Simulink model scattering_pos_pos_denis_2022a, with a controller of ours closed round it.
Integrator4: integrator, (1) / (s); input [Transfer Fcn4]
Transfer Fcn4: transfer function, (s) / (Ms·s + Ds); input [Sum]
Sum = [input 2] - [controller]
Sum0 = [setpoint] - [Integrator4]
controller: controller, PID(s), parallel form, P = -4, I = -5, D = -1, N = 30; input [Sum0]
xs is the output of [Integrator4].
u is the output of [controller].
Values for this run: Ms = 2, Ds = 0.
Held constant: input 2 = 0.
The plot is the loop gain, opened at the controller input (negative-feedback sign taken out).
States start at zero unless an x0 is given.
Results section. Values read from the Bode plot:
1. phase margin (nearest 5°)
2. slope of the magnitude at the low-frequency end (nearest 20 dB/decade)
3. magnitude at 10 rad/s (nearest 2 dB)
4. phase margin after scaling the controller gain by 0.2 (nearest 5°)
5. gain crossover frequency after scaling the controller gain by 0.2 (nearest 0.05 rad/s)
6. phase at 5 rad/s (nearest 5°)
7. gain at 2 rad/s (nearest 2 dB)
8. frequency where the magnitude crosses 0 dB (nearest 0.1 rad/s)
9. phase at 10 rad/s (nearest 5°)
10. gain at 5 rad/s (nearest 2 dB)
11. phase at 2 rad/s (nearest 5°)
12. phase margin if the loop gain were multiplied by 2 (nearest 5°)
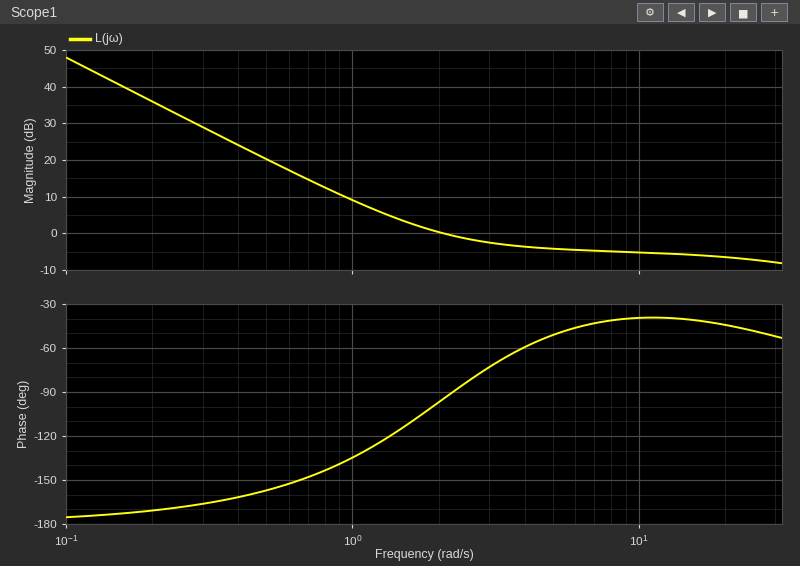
85°
-40 dB/decade
-6 dB
35°
0.75 rad/s
-50°
0 dB
2.1 rad/s
-40°
-4 dB
-95°
140°
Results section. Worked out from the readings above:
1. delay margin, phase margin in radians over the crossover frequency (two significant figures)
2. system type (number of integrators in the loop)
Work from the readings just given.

0.71 s
2
